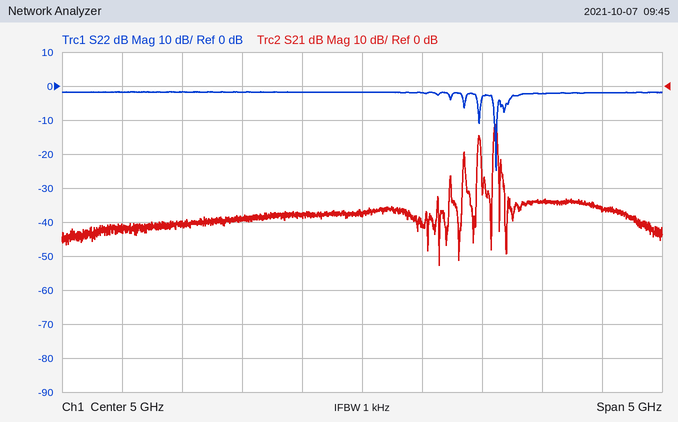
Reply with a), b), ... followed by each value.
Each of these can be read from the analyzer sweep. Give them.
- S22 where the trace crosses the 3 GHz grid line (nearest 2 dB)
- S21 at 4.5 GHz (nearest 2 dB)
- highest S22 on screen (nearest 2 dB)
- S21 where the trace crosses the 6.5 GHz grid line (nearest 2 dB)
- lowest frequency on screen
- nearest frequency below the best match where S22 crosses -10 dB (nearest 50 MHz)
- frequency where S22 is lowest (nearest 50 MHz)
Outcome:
a) -2 dB
b) -38 dB
c) -2 dB
d) -34 dB
e) 2.5 GHz
f) 6.10 GHz
g) 6.10 GHz
